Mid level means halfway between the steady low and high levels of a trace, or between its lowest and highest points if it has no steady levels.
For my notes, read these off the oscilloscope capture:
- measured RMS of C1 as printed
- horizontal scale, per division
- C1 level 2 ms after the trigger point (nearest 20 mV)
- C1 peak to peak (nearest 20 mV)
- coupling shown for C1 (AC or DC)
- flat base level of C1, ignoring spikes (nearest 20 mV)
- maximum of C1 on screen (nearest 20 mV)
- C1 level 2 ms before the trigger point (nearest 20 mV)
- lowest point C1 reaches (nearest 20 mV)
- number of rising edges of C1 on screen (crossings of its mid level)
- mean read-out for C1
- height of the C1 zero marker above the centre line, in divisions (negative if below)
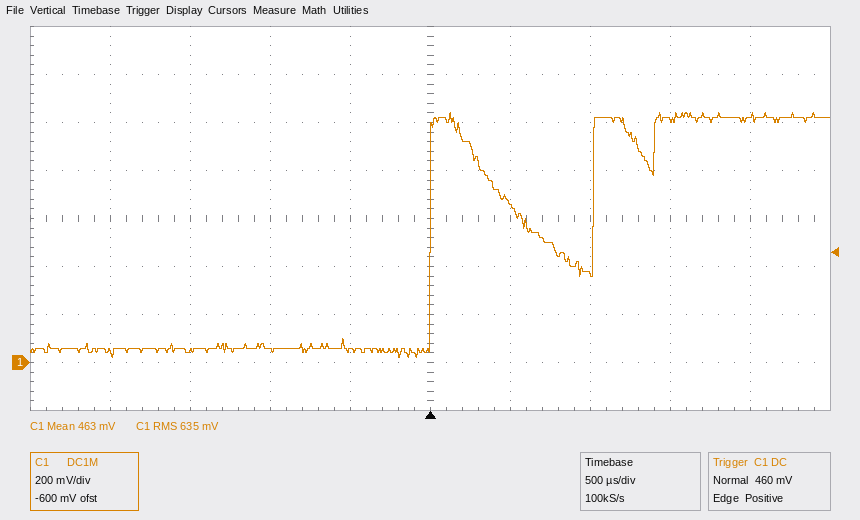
635 mV
500 µs
1.02 V
1.02 V
DC
60 mV
1.04 V
40 mV
20 mV
2
463 mV
-3.0 div
